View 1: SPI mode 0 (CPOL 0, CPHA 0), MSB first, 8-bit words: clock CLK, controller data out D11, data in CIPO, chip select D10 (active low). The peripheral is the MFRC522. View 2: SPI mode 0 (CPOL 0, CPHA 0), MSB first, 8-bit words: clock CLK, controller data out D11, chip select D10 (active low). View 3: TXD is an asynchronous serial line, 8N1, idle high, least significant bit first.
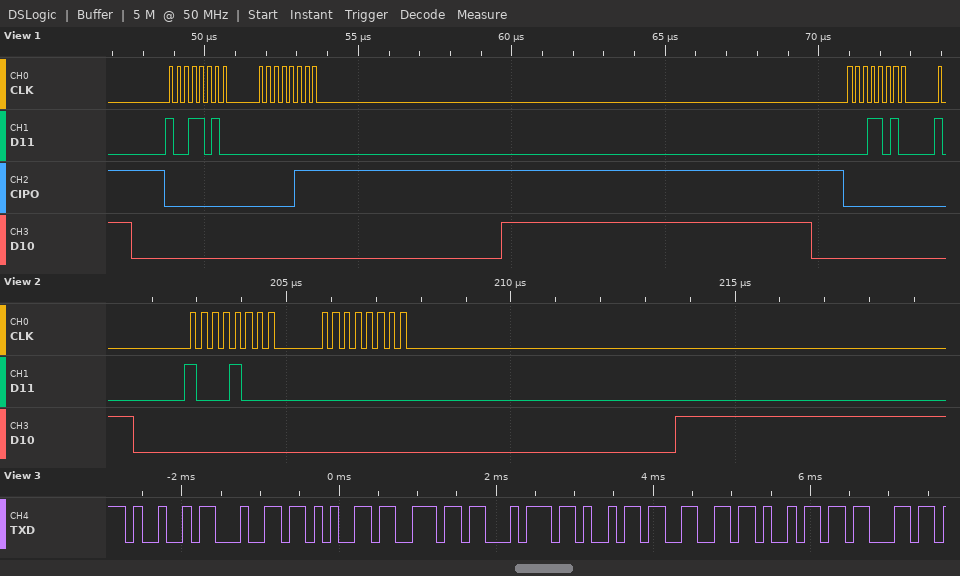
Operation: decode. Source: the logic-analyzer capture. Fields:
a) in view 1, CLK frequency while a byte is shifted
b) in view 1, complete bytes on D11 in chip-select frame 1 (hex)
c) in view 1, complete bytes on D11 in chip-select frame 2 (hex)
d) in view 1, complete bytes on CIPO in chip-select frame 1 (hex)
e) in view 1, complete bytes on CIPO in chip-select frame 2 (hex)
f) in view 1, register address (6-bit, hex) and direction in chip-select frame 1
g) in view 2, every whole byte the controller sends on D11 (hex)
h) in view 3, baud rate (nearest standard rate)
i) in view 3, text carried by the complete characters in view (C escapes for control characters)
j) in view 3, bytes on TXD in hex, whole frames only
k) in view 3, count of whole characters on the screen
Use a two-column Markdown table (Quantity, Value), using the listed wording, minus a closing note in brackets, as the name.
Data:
| Quantity | Value |
|---|---|
| in view 1, CLK frequency while a byte is shifted | 4 MHz |
| in view 1, complete bytes on D11 in chip-select frame 1 | 9A 00 |
| in view 1, complete bytes on D11 in chip-select frame 2 | 1A |
| in view 1, complete bytes on CIPO in chip-select frame 1 | 00 07 |
| in view 1, complete bytes on CIPO in chip-select frame 2 | 00 |
| in view 1, register address (6-bit, hex) and direction in chip-select frame 1 | 0x0D read |
| in view 2, every whole byte the controller sends on D11 | 88 00 |
| in view 3, baud rate | 9600 baud |
| in view 3, text carried by the complete characters in view | "Identific" |
| in view 3, bytes on TXD in hex, whole frames only | 49 64 65 6E 74 69 66 69 63 |
| in view 3, count of whole characters on the screen | 9 |
